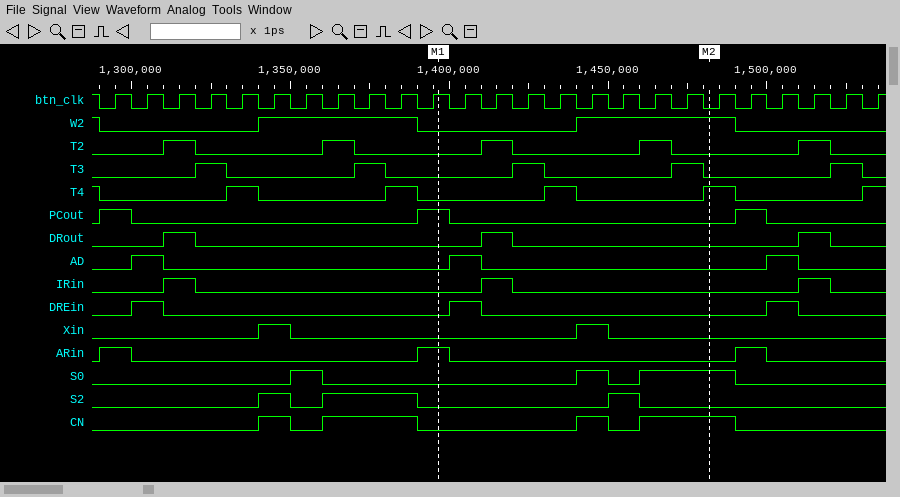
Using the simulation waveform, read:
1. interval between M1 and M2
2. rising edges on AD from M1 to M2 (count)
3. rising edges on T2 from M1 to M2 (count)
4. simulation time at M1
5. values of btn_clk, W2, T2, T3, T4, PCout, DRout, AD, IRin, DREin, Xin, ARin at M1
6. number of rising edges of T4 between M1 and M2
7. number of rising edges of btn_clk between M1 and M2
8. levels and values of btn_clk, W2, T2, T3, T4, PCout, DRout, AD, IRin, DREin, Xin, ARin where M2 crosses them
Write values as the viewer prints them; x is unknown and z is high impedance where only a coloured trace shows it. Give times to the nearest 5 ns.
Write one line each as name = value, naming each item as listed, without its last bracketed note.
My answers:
interval between M1 and M2 = 85 ns
rising edges on AD from M1 to M2 = 1
rising edges on T2 from M1 to M2 = 2
simulation time at M1 = 1395 ns
values of btn_clk, W2, T2, T3, T4, PCout, DRout, AD, IRin, DREin, Xin, ARin at M1 = btn_clk=1, W2=0, T2=0, T3=0, T4=0, PCout=1, DRout=0, AD=0, IRin=0, DREin=0, Xin=0, ARin=1
number of rising edges of T4 between M1 and M2 = 2
number of rising edges of btn_clk between M1 and M2 = 8
levels and values of btn_clk, W2, T2, T3, T4, PCout, DRout, AD, IRin, DREin, Xin, ARin where M2 crosses them = btn_clk=0, W2=1, T2=0, T3=0, T4=1, PCout=0, DRout=0, AD=0, IRin=0, DREin=0, Xin=0, ARin=0
